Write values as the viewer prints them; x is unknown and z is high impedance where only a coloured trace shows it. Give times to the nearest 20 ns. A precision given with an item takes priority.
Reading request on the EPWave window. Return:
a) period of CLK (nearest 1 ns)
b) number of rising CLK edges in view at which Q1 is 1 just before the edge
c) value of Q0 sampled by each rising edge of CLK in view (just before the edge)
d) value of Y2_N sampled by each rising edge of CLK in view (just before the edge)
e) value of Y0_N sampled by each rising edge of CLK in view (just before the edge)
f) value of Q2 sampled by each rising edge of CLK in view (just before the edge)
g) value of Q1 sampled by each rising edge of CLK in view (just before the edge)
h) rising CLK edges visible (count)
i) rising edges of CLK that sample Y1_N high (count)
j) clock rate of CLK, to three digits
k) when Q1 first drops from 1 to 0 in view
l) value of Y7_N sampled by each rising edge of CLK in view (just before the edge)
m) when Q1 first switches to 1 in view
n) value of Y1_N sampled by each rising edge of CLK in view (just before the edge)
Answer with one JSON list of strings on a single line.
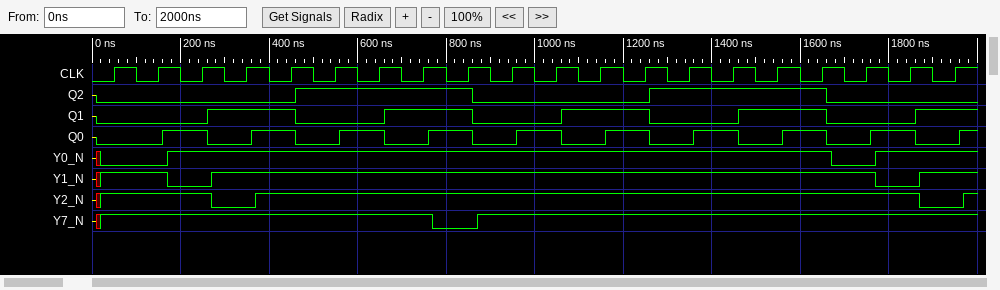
["100 ns", "9", "0 0 1 0 1 0 1 0 1 0 1 0 1 0 1 0 1 0 1 0", "1 1 1 0 1 1 1 1 1 1 1 1 1 1 1 1 1 1 1 0", "0 0 1 1 1 1 1 1 1 1 1 1 1 1 1 1 1 0 1 1", "0 0 0 0 0 1 1 1 1 0 0 0 0 1 1 1 1 0 0 0", "0 0 0 1 1 0 0 1 1 0 0 1 1 0 0 1 1 0 0 1", "20", "18", "10.0 MHz", "460 ns", "1 1 1 1 1 1 1 1 0 1 1 1 1 1 1 1 1 1 1 1", "260 ns", "1 1 0 1 1 1 1 1 1 1 1 1 1 1 1 1 1 1 0 1"]
